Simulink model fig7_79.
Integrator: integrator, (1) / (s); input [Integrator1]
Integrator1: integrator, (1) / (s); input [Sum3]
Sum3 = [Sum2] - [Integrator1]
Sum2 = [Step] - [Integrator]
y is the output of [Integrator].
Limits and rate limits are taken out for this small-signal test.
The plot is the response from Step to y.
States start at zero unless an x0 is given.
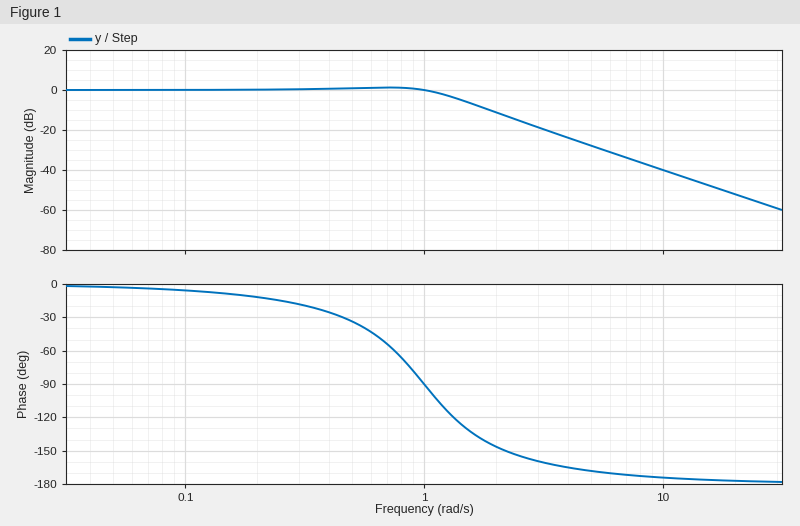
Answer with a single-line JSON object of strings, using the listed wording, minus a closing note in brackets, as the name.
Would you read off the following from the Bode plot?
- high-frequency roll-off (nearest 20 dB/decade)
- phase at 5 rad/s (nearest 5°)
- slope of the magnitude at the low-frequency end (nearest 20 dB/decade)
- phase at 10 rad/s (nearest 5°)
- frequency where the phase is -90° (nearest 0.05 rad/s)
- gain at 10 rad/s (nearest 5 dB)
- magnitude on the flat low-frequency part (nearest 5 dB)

{"high-frequency roll-off": "-40 dB/decade", "phase at 5 rad/s": "-170°", "slope of the magnitude at the low-frequency end": "0 dB/decade", "phase at 10 rad/s": "-175°", "frequency where the phase is -90°": "1.00 rad/s", "gain at 10 rad/s": "-40 dB", "magnitude on the flat low-frequency part": "0 dB"}
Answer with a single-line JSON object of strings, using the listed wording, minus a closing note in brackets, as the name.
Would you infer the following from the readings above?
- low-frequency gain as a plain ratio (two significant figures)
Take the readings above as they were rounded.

{"low-frequency gain as a plain ratio": "1.0"}
